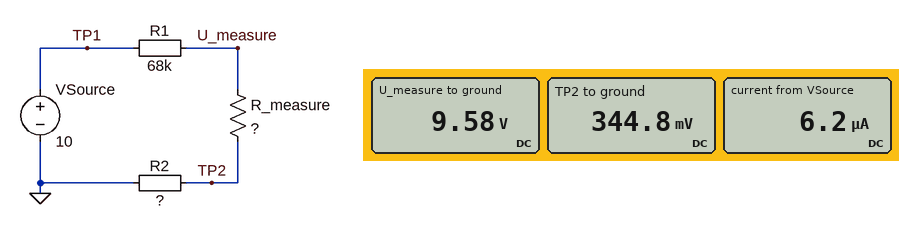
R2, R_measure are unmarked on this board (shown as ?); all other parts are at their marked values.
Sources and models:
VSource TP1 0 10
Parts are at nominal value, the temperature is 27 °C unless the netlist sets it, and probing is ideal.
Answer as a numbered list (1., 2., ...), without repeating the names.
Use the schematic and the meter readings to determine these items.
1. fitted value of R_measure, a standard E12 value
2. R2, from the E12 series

1. 1.5 MΩ
2. 56 kΩ
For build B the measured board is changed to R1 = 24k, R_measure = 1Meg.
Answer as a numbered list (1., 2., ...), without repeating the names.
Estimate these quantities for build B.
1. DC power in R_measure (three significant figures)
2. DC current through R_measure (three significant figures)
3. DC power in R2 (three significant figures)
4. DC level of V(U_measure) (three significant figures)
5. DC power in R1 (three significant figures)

1. 85.7 µW
2. 9.26 µA
3. 4.80 µW
4. 9.78 V
5. 2.06 µW
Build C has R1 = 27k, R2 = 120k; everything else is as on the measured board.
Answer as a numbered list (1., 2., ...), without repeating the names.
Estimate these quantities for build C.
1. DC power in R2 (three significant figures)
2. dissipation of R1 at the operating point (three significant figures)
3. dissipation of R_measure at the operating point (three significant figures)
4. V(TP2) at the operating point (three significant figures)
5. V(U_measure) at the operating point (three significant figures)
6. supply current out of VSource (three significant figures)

1. 4.42 µW
2. 995 nW
3. 55.3 µW
4. 729 mV
5. 9.84 V
6. 6.07 µA
